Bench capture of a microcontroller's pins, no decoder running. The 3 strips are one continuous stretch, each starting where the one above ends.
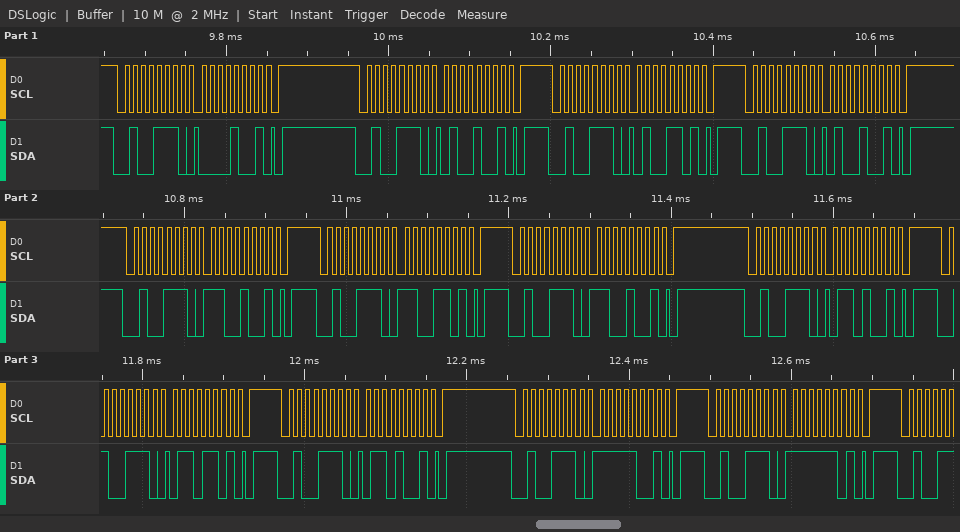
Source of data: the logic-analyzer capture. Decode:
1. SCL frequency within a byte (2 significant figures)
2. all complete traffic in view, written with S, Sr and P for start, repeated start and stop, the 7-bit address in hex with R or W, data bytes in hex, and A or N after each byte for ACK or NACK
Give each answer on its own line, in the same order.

100 kHz
S 27W A 09 A P S 27W A 49 A P S 27W A 4D A P S 27W A 49 A P S 27W A C9 A P S 27W A CD A P S 27W A C9 A P S 27W A 69 A P S 27W A 6D A P S 27W A 69 A P S 27W A F9 A P S 27W A FD A P
